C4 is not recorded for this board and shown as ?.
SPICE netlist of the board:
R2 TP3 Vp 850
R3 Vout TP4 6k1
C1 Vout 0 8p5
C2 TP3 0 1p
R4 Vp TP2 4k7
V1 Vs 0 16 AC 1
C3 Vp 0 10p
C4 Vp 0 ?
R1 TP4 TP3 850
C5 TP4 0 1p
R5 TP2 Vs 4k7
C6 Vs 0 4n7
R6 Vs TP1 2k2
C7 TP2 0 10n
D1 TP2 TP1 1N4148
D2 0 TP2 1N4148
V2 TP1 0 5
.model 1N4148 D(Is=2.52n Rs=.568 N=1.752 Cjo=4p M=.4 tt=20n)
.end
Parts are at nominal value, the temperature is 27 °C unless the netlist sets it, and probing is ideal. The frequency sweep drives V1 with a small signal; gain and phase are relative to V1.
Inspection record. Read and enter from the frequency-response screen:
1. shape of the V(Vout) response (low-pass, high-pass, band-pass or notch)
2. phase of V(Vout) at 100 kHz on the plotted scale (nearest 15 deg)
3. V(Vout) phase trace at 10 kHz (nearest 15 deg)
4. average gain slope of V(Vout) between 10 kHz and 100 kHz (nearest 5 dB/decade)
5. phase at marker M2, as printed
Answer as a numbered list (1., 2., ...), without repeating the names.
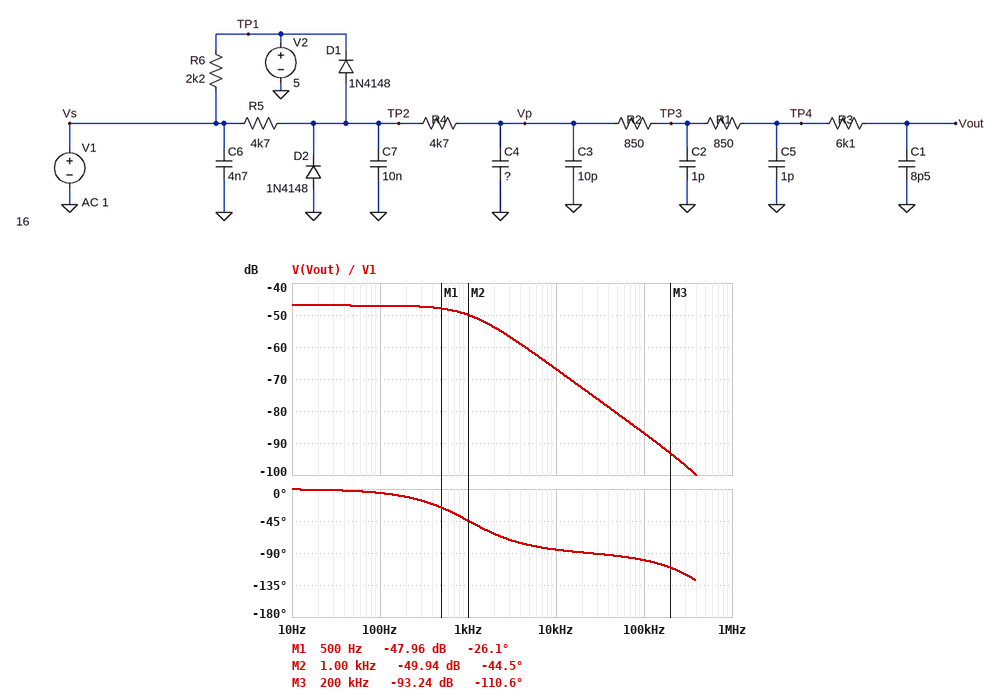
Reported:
1. low-pass
2. -105 deg
3. -90 deg
4. -20 dB/decade
5. -44.5 deg
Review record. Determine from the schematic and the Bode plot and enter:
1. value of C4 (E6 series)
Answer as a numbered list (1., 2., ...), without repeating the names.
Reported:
1. 33 nF
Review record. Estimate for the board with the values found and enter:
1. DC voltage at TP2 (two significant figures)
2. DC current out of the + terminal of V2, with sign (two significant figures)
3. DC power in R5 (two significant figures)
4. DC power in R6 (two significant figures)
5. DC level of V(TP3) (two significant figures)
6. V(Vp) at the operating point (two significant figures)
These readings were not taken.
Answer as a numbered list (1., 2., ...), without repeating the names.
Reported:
1. 5.6 V
2. -7.2 mA
3. 23 mW
4. 55 mW
5. 5.6 V
6. 5.6 V
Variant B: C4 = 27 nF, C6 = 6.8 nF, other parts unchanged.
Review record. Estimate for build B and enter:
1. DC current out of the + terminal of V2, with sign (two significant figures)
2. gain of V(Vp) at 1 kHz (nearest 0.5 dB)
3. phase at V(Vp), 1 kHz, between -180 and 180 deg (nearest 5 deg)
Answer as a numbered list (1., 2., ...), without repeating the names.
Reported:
1. -7.2 mA
2. -49.0 dB
3. -40 deg
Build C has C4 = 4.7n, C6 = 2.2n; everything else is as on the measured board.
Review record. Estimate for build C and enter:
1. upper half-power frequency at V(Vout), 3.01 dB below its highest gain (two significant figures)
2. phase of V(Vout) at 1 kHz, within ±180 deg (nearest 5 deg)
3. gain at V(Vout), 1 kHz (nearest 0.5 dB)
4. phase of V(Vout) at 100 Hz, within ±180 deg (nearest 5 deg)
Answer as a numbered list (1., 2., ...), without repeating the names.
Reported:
1. 7.1 kHz
2. -10 deg
3. -47.0 dB
4. 0 deg
